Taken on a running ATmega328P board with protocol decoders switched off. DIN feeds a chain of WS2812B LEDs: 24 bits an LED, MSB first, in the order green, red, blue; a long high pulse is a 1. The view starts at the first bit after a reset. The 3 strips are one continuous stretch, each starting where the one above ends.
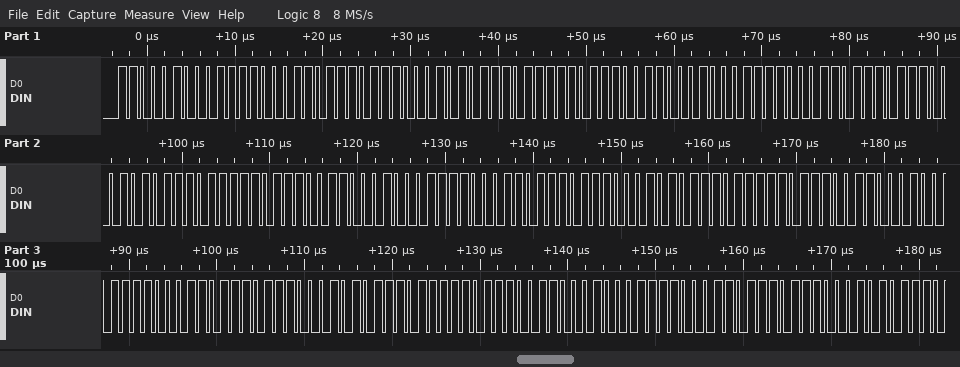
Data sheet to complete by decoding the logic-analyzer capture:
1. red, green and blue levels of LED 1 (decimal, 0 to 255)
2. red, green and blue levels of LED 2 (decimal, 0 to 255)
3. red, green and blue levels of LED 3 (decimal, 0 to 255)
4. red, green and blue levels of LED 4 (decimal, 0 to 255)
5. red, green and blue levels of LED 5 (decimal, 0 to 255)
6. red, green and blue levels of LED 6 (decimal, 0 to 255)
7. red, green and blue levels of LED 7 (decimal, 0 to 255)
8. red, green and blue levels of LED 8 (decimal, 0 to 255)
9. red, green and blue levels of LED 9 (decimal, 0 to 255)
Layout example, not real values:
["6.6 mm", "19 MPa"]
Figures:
["120, 196, 221", "119, 197, 220", "120, 196, 221", "119, 197, 220", "120, 196, 221", "119, 197, 220", "120, 196, 221", "119, 197, 220", "120, 196, 221"]
